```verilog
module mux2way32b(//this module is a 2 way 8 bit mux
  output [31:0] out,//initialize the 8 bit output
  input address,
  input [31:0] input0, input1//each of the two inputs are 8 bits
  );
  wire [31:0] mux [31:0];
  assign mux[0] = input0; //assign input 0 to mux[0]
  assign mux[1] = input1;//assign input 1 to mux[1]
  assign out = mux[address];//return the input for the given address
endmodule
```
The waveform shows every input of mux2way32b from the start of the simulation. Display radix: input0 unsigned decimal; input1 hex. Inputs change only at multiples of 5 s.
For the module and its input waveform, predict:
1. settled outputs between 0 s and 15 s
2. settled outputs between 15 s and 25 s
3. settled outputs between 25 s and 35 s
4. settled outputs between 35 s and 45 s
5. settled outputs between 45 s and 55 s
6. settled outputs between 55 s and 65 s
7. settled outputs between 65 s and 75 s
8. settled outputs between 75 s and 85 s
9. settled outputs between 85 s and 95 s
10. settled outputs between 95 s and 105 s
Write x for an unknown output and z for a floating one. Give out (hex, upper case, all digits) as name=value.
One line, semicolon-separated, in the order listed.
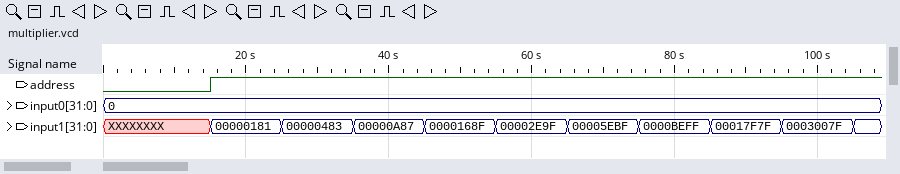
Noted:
out=00000000; out=00000181; out=00000483; out=00000A87; out=0000168F; out=00002E9F; out=00005EBF; out=0000BEFF; out=00017F7F; out=0003007F
